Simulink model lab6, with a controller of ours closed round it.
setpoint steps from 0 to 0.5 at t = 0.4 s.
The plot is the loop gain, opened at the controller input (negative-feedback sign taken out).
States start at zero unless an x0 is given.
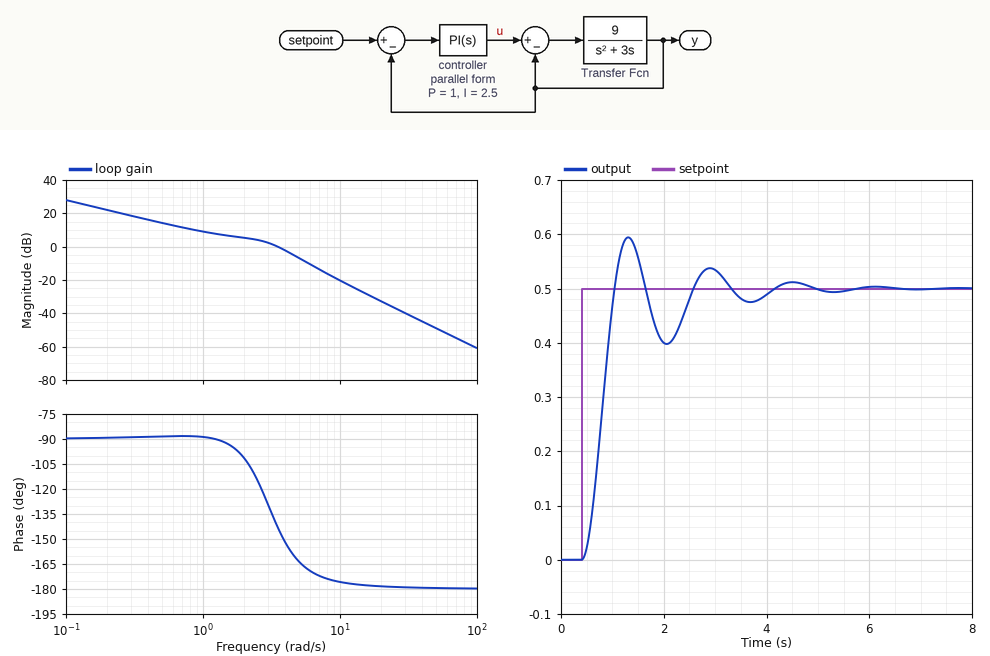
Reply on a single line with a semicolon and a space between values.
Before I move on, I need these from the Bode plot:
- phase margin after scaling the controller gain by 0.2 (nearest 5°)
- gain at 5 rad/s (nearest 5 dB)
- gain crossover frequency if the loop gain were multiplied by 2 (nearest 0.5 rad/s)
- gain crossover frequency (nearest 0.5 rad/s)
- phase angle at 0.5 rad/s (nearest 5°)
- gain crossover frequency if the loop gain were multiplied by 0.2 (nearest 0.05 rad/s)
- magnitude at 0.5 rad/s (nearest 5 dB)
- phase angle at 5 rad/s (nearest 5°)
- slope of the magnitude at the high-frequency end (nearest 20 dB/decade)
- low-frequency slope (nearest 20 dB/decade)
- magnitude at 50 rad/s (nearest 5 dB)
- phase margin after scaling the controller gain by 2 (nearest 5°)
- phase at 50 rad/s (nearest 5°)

90°; -5 dB; 5.0 rad/s; 3.5 rad/s; -90°; 0.50 rad/s; 15 dB; -165°; -40 dB/decade; -20 dB/decade; -50 dB; 20°; -180°
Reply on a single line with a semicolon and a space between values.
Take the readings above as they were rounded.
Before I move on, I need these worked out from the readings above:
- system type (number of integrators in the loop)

1
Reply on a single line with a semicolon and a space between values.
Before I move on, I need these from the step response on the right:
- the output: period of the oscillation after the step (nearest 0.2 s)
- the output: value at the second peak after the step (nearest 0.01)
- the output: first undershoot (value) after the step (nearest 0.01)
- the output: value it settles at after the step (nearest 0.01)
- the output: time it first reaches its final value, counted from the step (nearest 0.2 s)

1.6 s; 0.54; 0.40; 0.50; 0.6 s
